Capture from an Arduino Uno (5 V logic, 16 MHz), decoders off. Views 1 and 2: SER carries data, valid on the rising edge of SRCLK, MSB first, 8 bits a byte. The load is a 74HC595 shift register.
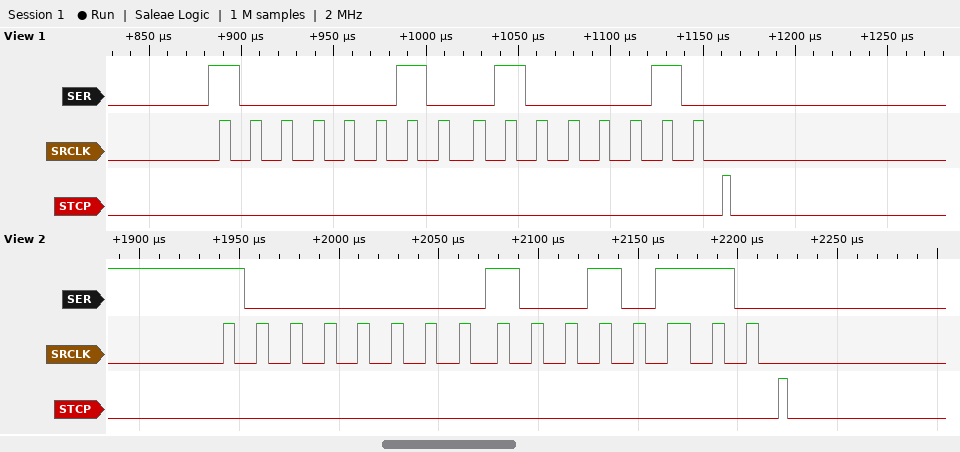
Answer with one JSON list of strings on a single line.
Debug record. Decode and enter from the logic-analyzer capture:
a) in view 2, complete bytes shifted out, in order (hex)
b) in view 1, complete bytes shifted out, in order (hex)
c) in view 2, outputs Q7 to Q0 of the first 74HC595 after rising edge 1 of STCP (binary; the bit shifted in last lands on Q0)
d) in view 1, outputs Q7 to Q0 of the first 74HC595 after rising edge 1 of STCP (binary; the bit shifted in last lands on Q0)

["80 96", "82 42", "10010110", "01000010"]
